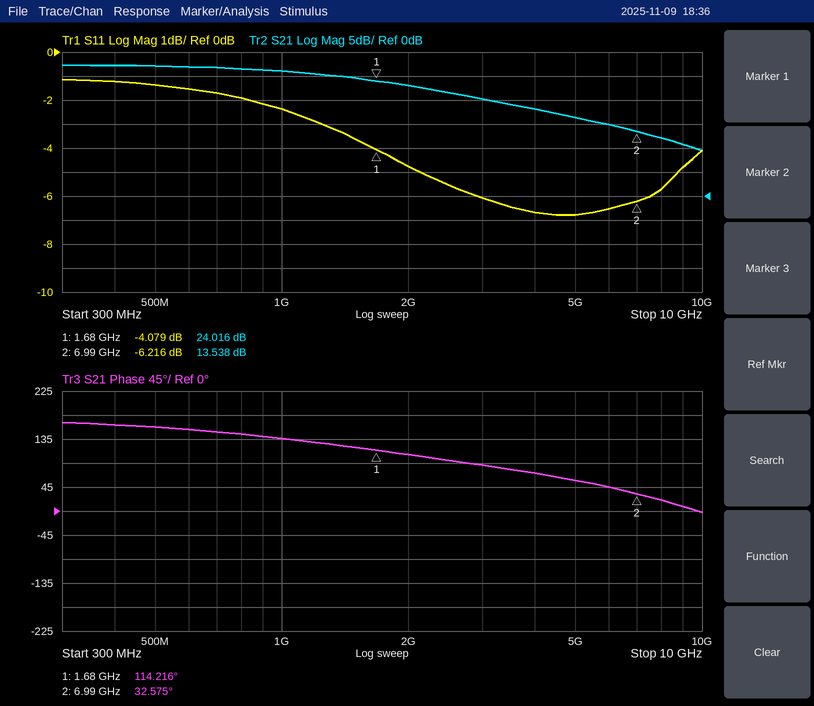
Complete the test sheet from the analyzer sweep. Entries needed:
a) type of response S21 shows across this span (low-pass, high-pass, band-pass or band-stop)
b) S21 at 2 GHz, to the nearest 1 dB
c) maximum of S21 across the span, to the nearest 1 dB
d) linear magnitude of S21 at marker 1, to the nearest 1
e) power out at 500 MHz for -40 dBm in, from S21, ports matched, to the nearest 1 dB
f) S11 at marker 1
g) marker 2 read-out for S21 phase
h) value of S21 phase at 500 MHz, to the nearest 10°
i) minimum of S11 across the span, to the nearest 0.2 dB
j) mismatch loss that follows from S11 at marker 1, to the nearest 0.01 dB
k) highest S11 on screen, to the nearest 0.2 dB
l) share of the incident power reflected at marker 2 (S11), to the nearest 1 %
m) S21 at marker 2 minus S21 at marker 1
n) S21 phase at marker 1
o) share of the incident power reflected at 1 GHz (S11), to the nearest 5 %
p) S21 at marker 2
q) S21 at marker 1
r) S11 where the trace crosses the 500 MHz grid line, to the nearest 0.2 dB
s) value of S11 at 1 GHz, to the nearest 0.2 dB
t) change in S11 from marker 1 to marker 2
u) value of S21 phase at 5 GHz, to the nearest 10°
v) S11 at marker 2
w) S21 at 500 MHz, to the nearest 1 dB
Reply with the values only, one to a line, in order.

low-pass
23 dB
27 dB
16
-13 dBm
-4.079 dB
32.575°
160°
-6.8 dB
2.15 dB
-1.2 dB
24 %
-10.478 dB
114.216°
60 %
13.538 dB
24.016 dB
-1.4 dB
-2.4 dB
-2.137 dB
60°
-6.216 dB
27 dB
